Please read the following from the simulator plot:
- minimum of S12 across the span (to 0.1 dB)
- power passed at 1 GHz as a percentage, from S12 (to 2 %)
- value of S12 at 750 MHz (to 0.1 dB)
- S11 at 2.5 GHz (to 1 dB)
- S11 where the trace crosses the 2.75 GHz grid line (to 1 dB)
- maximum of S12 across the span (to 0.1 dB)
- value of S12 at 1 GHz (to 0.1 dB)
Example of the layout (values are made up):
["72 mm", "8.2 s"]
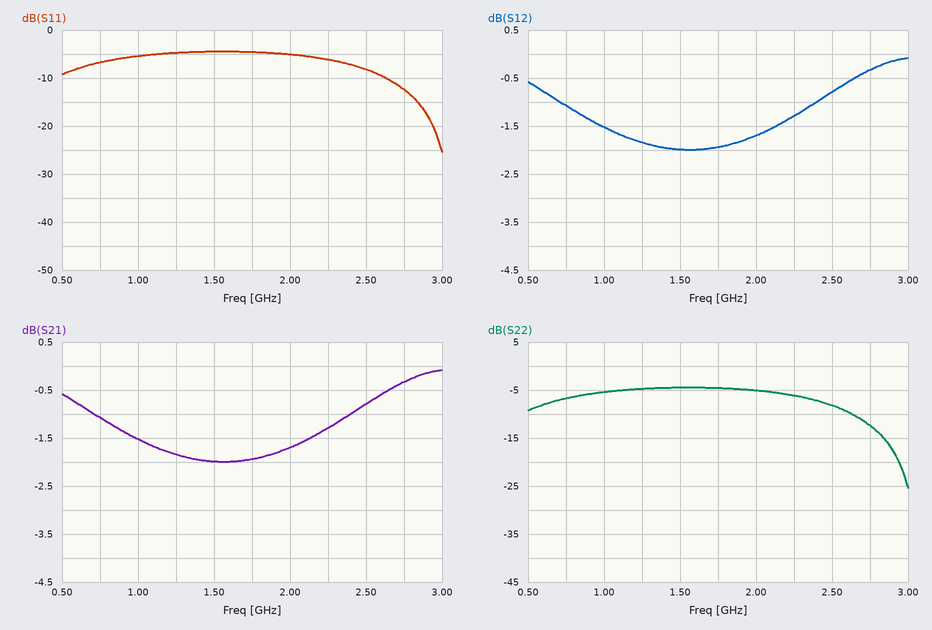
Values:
["-2.0 dB", "70 %", "-1.1 dB", "-8 dB", "-12 dB", "-0.1 dB", "-1.5 dB"]
